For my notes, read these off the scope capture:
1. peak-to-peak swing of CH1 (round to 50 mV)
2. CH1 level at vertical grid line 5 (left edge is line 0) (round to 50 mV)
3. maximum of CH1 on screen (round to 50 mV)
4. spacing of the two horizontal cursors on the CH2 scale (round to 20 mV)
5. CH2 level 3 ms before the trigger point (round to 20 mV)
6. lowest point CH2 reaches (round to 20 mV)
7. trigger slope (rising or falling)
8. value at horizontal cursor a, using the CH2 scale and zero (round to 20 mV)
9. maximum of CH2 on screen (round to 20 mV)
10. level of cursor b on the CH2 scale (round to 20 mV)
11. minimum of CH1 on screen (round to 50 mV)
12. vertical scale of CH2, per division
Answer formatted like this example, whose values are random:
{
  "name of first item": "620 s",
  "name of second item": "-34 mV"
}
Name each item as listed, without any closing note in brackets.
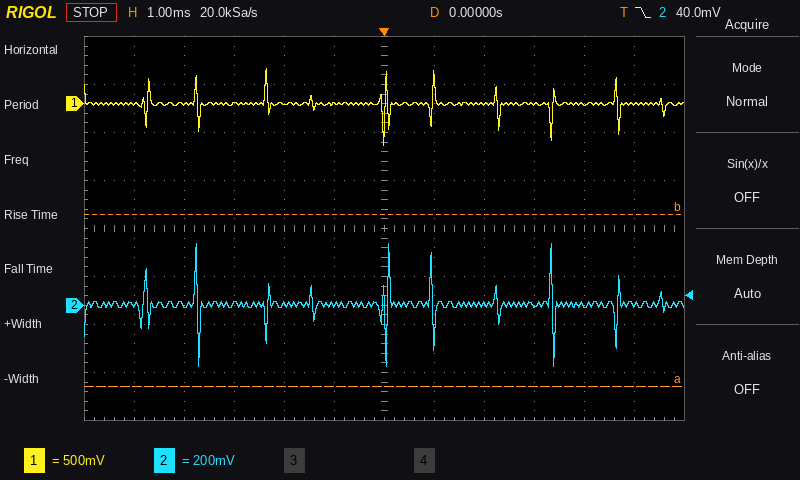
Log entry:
{
  "peak-to-peak swing of CH1": "800 mV",
  "CH1 level at vertical grid line 5 (left edge is line 0)": "0 mV",
  "maximum of CH1 on screen": "350 mV",
  "spacing of the two horizontal cursors on the CH2 scale": "720 mV",
  "CH2 level 3 ms before the trigger point": "0 mV",
  "lowest point CH2 reaches": "-260 mV",
  "trigger slope": "falling",
  "value at horizontal cursor a, using the CH2 scale and zero": "-340 mV",
  "maximum of CH2 on screen": "260 mV",
  "level of cursor b on the CH2 scale": "380 mV",
  "minimum of CH1 on screen": "-450 mV",
  "vertical scale of CH2, per division": "200 mV"
}
